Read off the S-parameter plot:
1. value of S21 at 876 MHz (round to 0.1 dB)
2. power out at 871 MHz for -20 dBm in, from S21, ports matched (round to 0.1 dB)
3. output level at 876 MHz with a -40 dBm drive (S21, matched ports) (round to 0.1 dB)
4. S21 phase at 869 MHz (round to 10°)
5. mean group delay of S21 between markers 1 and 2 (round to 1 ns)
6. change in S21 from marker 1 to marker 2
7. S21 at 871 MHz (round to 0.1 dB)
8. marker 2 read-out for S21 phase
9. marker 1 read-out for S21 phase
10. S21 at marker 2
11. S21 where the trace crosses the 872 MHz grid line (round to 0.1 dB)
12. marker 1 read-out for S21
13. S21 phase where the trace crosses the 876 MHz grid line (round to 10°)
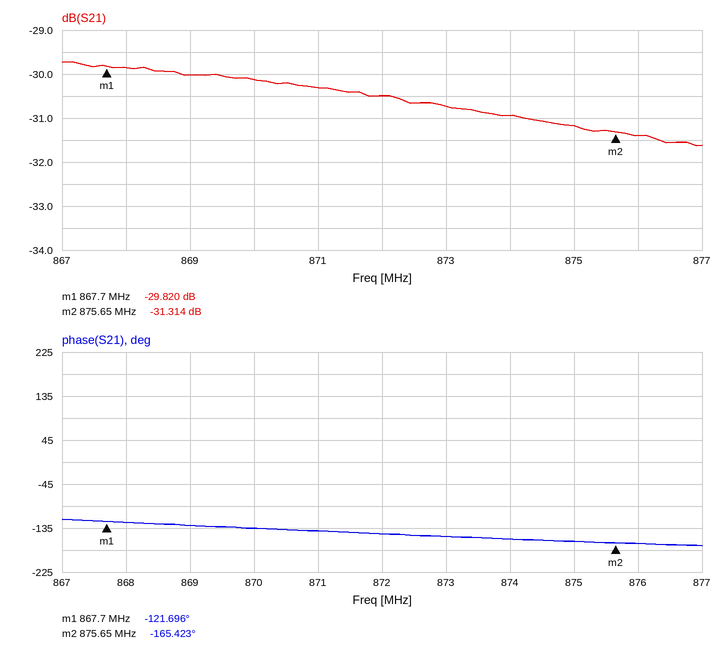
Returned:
-31.4 dB
-50.3 dBm
-71.4 dBm
-130°
15 ns
-1.494 dB
-30.3 dB
-165.423°
-121.696°
-31.314 dB
-30.5 dB
-29.820 dB
-170°
